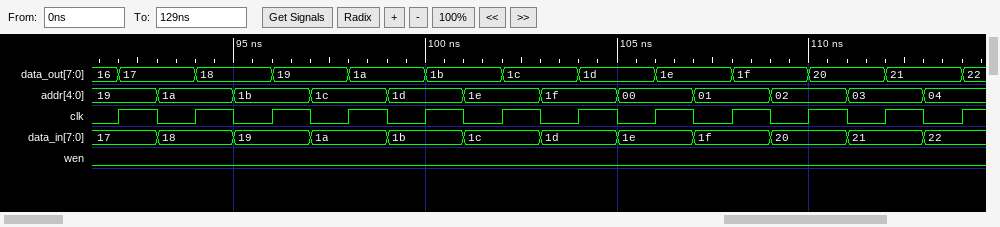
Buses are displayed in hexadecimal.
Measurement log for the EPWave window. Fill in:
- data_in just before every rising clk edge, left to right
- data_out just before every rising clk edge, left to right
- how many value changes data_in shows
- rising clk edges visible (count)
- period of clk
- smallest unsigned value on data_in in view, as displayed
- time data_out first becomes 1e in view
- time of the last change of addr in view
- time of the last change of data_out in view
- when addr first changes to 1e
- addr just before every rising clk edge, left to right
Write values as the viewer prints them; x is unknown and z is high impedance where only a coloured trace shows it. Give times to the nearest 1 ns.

17, 18, 19, 1a, 1b, 1c, 1d, 1e, 1f, 20, 21, 22
16, 17, 18, 19, 1a, 1b, 1c, 1d, 1e, 1f, 20, 21
11
12
2 ns
17
106 ns
113 ns
114 ns
101 ns
19, 1a, 1b, 1c, 1d, 1e, 1f, 00, 01, 02, 03, 04
